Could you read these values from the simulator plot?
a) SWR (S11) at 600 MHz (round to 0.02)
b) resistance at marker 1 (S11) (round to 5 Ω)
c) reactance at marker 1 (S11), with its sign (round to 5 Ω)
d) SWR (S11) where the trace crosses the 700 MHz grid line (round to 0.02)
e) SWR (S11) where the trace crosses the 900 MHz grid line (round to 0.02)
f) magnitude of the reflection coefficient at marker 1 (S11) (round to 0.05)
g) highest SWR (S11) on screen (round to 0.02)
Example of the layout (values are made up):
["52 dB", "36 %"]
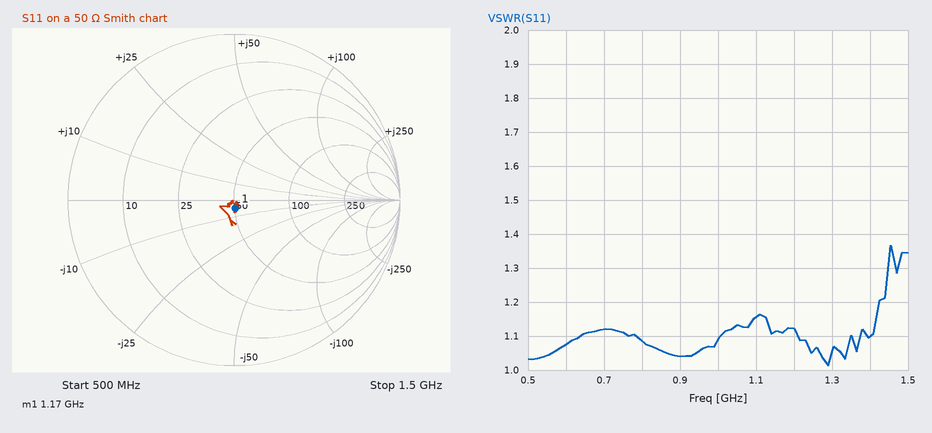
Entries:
["1.08", "50 Ω", "-5 Ω", "1.12", "1.04", "0.05", "1.36"]
